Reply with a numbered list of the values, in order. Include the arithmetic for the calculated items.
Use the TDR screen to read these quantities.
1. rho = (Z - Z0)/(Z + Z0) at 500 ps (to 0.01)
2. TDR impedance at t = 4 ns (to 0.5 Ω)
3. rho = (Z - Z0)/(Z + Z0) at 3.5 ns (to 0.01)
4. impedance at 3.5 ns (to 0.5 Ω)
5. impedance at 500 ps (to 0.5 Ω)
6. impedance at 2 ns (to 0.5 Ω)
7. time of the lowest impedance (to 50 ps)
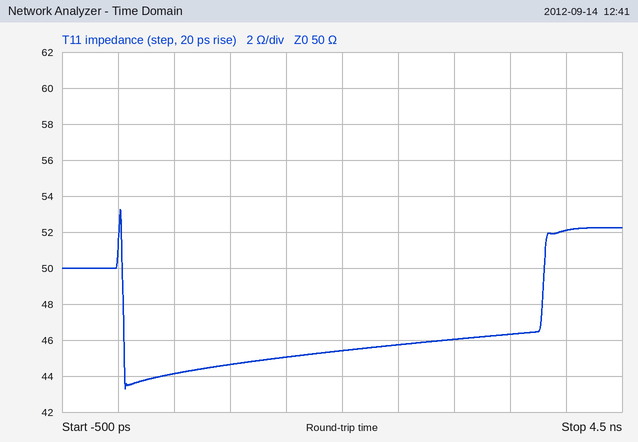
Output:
1. (44 − 50)/(44 + 50) ≈ -0.06
2. 52.0 Ω
3. (46.5 − 50)/(46.5 + 50) ≈ -0.04
4. 46.5 Ω
5. 44.0 Ω
6. 45.5 Ω
7. 50 ps
